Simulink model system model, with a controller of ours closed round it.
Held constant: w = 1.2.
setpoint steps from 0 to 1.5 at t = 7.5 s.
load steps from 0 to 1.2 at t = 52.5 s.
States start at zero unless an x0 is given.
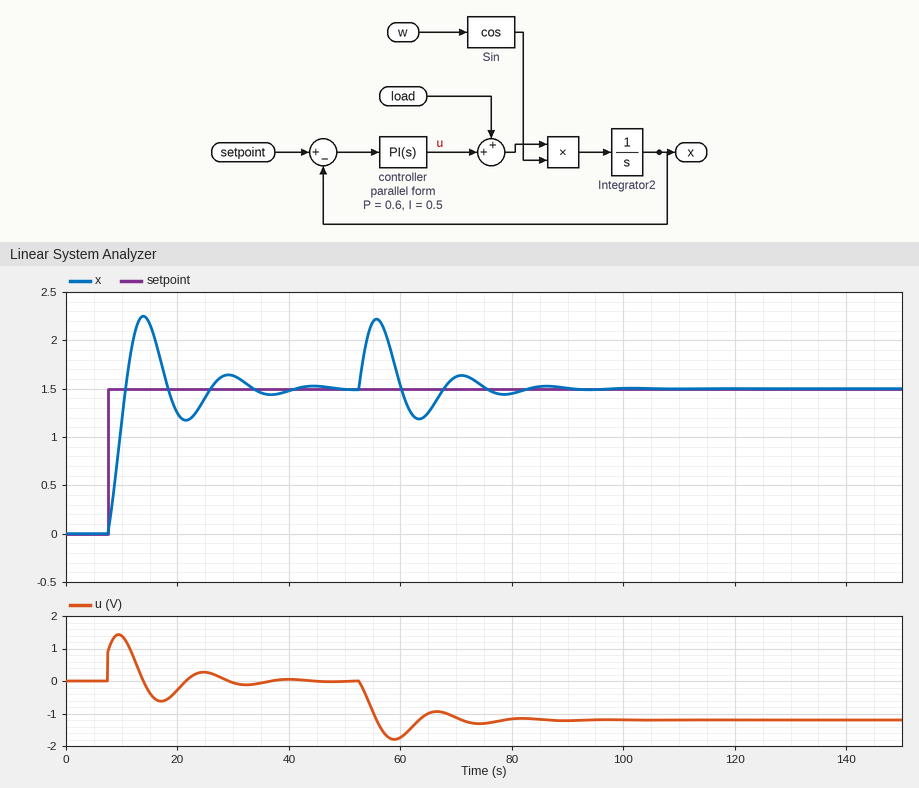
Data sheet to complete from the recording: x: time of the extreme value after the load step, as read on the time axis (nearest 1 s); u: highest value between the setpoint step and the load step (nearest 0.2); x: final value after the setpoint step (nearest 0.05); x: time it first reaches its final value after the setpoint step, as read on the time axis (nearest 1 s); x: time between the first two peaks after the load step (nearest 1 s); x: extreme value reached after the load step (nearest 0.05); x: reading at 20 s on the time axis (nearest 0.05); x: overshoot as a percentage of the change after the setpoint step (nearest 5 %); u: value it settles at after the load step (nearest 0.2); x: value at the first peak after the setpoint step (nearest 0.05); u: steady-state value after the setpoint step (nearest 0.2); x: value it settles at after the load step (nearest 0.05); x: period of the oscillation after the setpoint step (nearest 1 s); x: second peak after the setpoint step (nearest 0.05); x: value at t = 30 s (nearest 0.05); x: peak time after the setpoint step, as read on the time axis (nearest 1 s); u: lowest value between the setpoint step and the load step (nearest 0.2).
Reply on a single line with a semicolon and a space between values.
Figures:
56 s; 1.4; 1.50; 11 s; 15 s; 2.20; 1.25; 50 %; -1.2; 2.25; 0.0; 1.50; 15 s; 1.65; 1.65; 14 s; -0.6
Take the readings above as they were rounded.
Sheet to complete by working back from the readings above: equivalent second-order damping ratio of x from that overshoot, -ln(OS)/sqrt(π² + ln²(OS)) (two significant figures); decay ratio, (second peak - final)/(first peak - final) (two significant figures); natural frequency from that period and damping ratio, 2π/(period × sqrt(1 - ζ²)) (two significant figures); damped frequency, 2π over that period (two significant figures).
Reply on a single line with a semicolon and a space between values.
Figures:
0.22; 0.20; 0.43 rad/s; 0.42 rad/s
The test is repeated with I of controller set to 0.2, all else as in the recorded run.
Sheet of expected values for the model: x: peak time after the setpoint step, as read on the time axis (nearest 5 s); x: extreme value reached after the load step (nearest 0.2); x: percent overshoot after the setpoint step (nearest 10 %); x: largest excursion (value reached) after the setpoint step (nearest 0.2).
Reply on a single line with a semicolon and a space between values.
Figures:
15 s; 2.4; 40 %; 2.0
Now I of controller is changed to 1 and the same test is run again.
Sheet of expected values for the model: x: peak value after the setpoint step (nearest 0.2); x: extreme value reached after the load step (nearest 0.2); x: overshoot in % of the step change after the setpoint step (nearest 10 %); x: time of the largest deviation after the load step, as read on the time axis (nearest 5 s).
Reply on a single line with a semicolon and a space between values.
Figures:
2.4; 2.0; 60 %; 55 s
